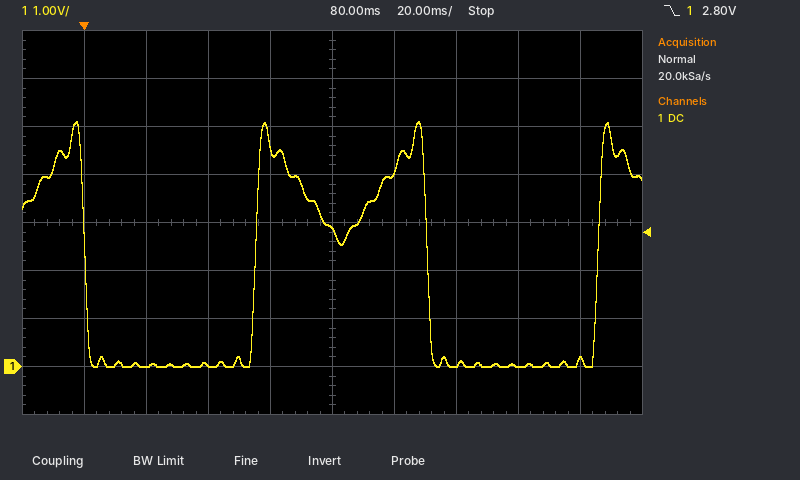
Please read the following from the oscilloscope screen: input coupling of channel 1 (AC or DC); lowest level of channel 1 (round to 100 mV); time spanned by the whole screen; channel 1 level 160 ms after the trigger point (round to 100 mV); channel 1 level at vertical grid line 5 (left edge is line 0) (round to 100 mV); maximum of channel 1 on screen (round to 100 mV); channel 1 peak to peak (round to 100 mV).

DC
0.0 V
200 ms
100 mV
2.9 V
5.1 V
5.1 V
